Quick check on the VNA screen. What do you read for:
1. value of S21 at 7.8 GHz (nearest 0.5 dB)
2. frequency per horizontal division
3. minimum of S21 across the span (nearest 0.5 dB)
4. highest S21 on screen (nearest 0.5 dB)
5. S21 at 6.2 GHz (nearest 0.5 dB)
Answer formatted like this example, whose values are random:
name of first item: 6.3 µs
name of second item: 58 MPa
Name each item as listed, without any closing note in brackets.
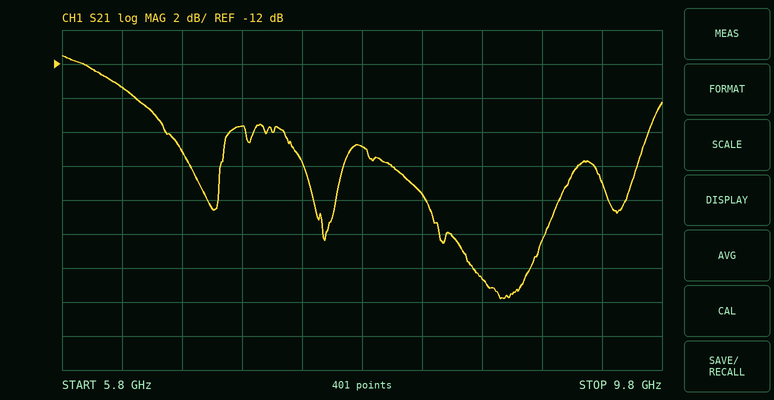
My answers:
value of S21 at 7.8 GHz: -17.0 dB
frequency per horizontal division: 400 MHz
minimum of S21 across the span: -26.0 dB
highest S21 on screen: -11.5 dB
S21 at 6.2 GHz: -13.5 dB
